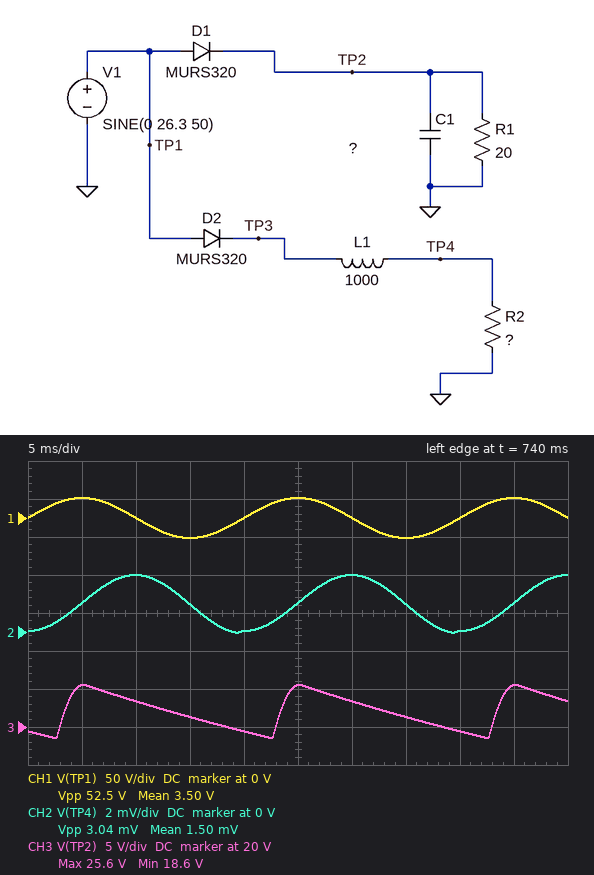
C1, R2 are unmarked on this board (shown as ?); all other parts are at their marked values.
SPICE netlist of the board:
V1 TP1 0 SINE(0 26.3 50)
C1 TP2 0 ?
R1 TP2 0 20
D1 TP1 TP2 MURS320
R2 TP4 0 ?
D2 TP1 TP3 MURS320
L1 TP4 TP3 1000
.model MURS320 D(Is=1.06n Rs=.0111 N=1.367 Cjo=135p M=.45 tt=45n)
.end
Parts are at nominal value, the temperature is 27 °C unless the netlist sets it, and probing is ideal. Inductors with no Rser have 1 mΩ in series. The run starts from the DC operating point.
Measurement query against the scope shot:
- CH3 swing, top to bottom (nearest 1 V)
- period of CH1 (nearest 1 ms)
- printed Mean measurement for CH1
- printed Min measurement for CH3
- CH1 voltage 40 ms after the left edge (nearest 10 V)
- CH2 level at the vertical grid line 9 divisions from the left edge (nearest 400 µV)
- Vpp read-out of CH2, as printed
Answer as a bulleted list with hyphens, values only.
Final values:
- 7 V
- 20 ms
- 3.50 V
- 18.6 V
- 0 V
- 1.6 mV
- 3.04 mV
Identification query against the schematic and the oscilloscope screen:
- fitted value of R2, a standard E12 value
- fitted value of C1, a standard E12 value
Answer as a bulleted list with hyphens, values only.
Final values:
- 18 Ω
- 2.7 mF
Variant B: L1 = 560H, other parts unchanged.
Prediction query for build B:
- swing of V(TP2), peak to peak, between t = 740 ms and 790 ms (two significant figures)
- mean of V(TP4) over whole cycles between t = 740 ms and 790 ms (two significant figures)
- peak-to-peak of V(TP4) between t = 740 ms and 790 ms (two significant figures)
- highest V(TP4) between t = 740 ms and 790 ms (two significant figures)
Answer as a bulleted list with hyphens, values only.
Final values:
- 7.0 V
- 2.6 mV
- 5.4 mV
- 5.3 mV
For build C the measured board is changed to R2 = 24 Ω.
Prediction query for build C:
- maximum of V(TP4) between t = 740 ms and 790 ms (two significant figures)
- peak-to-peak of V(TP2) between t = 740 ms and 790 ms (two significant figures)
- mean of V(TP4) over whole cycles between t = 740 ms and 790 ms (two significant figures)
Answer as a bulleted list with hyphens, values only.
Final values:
- 4.0 mV
- 7.0 V
- 2.0 mV
